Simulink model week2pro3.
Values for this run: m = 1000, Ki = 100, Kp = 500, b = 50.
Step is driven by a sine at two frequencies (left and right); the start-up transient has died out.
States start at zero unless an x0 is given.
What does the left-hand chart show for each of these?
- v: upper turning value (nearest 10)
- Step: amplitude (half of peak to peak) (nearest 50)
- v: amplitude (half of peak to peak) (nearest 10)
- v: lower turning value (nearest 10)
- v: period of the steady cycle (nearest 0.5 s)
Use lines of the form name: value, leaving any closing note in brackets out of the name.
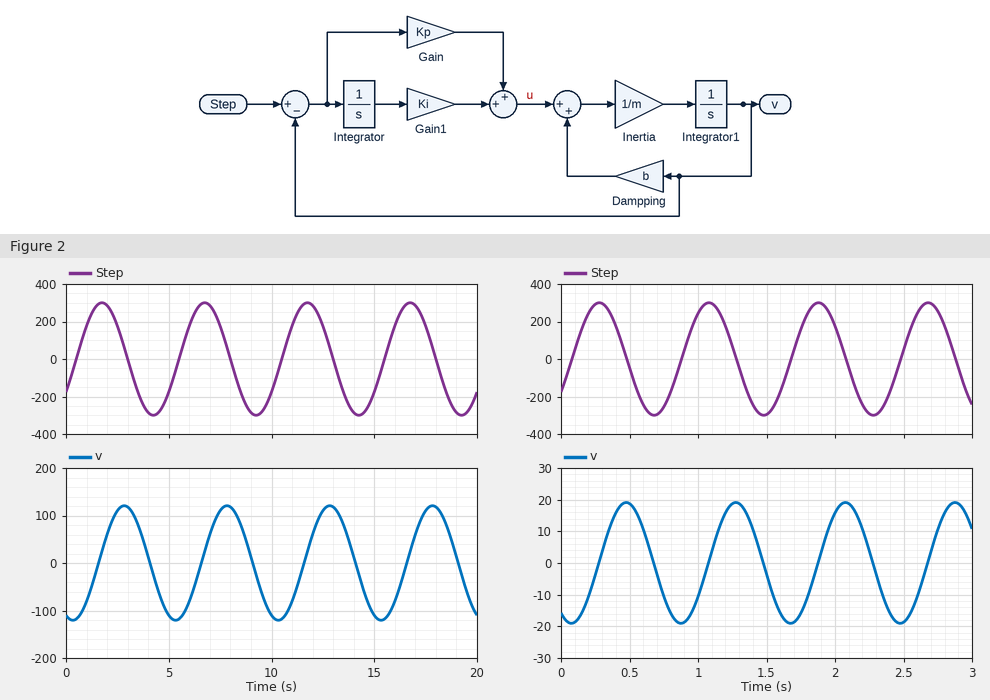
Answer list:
v: upper turning value: 120
Step: amplitude (half of peak to peak): 300
v: amplitude (half of peak to peak): 120
v: lower turning value: -120
v: period of the steady cycle: 5.0 s
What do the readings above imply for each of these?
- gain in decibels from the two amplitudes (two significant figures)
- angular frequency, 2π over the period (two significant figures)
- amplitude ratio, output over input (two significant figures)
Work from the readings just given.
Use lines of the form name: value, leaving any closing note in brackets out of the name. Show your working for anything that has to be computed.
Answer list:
gain in decibels from the two amplitudes: 20 log10(120 / 300) = -8.0 dB
angular frequency, 2π over the period: 2π / 5 = 1.3 rad/s
amplitude ratio, output over input: 120 / 300 = 0.40
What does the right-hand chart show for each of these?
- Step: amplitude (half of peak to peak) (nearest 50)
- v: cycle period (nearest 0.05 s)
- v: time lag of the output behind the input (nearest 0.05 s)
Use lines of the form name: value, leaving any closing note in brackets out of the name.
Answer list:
Step: amplitude (half of peak to peak): 300
v: cycle period: 0.80 s
v: time lag of the output behind the input: 0.20 s
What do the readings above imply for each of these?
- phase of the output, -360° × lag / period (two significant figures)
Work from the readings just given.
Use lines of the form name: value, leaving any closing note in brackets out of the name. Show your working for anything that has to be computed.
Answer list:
phase of the output, -360° × lag / period: -360 × 0.2 / 0.8 = -90°
